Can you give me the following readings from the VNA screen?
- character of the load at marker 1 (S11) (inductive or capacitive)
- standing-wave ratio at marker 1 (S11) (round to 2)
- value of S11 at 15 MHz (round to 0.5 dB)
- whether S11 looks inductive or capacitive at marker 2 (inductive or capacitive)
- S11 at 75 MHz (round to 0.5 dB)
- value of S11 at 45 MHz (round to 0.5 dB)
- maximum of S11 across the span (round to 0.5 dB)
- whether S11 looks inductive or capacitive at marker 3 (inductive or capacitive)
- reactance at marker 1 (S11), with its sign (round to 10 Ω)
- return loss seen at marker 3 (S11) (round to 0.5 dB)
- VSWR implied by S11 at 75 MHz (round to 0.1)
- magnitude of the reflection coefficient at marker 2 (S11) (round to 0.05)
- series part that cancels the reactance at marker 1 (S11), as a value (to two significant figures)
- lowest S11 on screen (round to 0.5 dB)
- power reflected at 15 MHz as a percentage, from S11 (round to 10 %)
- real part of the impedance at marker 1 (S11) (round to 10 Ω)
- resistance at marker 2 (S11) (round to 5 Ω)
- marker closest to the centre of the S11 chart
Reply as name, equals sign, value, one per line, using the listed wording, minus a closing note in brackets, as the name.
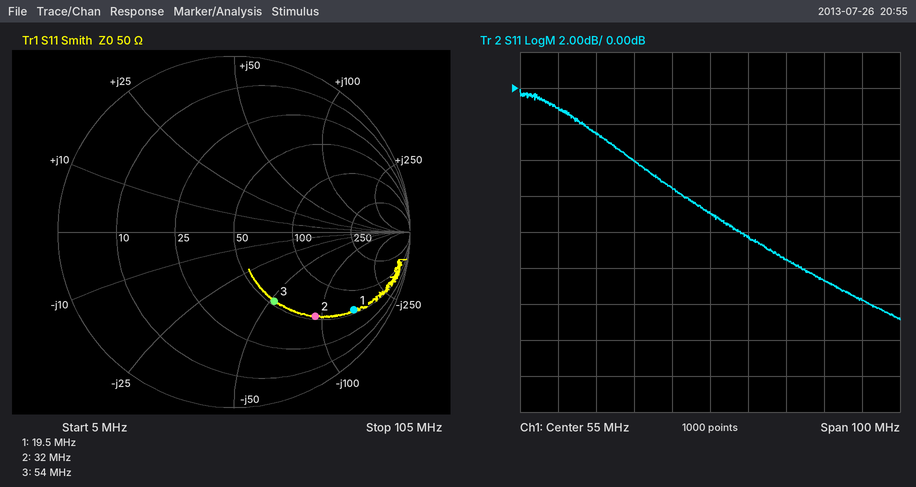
character of the load at marker 1 (S11) = capacitive
standing-wave ratio at marker 1 (S11) = 10
value of S11 at 15 MHz = -1.0 dB
whether S11 looks inductive or capacitive at marker 2 = capacitive
S11 at 75 MHz = -9.5 dB
value of S11 at 45 MHz = -5.5 dB
maximum of S11 across the span = 0.0 dB
whether S11 looks inductive or capacitive at marker 3 = capacitive
reactance at marker 1 (S11), with its sign = -150 Ω
return loss seen at marker 3 (S11) = 7.0 dB
VSWR implied by S11 at 75 MHz = 2.0
magnitude of the reflection coefficient at marker 2 (S11) = 0.65
series part that cancels the reactance at marker 1 (S11), as a value = 1.2 µH
lowest S11 on screen = -13.0 dB
power reflected at 15 MHz as a percentage, from S11 = 80 %
real part of the impedance at marker 1 (S11) = 60 Ω
resistance at marker 2 (S11) = 55 Ω
marker closest to the centre of the S11 chart = marker 3
